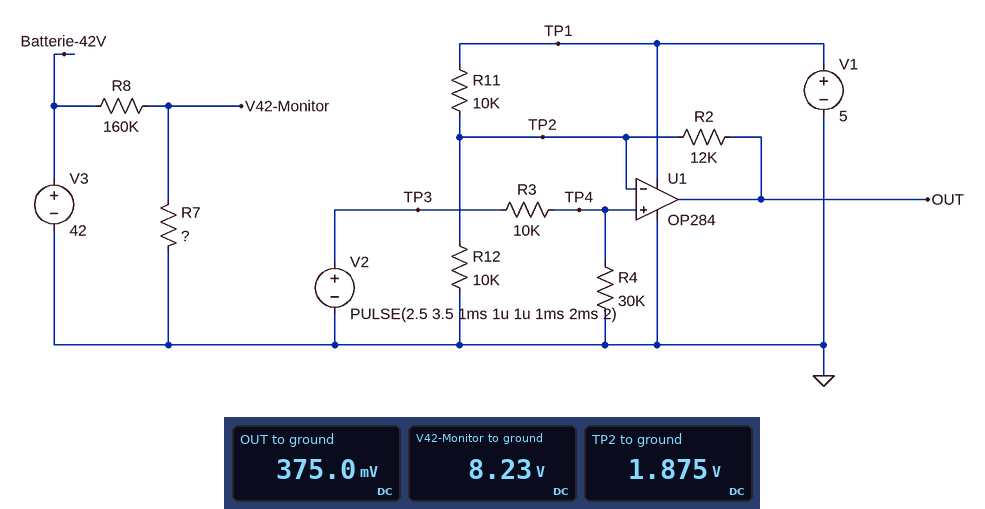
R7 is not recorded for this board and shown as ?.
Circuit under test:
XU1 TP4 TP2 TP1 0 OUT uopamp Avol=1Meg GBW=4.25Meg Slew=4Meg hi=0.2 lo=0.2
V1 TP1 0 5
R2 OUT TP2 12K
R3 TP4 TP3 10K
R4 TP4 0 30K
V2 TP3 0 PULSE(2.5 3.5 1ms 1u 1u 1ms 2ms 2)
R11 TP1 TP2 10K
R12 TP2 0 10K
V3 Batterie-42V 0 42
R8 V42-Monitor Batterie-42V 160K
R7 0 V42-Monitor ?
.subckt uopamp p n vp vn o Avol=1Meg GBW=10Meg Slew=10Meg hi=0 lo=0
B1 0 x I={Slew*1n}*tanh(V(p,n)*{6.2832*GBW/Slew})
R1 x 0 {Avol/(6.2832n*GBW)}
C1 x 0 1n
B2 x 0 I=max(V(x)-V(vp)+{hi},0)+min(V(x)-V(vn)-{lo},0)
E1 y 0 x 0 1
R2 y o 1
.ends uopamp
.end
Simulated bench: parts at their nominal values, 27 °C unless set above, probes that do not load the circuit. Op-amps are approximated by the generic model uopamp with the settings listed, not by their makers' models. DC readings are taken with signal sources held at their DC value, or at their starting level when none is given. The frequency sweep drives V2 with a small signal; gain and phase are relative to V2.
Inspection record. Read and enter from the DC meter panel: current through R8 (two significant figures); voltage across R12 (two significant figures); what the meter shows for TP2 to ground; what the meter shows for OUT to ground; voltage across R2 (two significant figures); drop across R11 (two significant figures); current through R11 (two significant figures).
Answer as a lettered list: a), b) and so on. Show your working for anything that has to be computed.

a) (42 V - 8.23 V) / 160 kΩ = 210 µA
b) 1.875 V = 1.9 V
c) 1.875 V
d) 375.0 mV
e) 1.875 V - 375 mV = 1.5 V
f) 5 V - 1.875 V = 3.1 V
g) (5 V - 1.875 V) / 10 kΩ = 310 µA
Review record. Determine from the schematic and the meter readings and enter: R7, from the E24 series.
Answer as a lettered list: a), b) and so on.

a) 39 kΩ
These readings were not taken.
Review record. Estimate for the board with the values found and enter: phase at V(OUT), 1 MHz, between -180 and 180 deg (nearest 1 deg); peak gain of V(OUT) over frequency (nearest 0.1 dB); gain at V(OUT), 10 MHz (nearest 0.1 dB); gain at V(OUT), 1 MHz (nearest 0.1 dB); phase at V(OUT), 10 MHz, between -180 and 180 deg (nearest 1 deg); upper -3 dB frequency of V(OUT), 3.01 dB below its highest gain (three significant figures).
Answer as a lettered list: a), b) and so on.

a) -39 deg
b) 8.1 dB
c) -10.0 dB
d) 6.0 dB
e) -83 deg
f) 1.25 MHz
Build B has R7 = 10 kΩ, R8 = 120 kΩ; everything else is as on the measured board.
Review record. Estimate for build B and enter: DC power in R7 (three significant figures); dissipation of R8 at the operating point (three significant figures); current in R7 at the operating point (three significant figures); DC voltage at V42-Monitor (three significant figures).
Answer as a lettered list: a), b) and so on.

a) 1.04 mW
b) 12.5 mW
c) 323 µA
d) 3.23 V
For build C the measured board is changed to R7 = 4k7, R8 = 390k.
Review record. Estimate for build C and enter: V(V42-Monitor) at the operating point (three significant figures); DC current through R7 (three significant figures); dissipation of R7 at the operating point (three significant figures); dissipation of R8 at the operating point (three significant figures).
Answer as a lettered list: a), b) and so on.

a) 500 mV
b) 106 µA
c) 53.2 µW
d) 4.42 mW
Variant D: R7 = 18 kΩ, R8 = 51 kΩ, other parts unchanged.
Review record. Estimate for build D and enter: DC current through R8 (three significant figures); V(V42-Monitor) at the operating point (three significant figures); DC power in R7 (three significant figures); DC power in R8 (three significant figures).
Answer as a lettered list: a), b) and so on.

a) 609 µA
b) 11.0 V
c) 6.67 mW
d) 18.9 mW
